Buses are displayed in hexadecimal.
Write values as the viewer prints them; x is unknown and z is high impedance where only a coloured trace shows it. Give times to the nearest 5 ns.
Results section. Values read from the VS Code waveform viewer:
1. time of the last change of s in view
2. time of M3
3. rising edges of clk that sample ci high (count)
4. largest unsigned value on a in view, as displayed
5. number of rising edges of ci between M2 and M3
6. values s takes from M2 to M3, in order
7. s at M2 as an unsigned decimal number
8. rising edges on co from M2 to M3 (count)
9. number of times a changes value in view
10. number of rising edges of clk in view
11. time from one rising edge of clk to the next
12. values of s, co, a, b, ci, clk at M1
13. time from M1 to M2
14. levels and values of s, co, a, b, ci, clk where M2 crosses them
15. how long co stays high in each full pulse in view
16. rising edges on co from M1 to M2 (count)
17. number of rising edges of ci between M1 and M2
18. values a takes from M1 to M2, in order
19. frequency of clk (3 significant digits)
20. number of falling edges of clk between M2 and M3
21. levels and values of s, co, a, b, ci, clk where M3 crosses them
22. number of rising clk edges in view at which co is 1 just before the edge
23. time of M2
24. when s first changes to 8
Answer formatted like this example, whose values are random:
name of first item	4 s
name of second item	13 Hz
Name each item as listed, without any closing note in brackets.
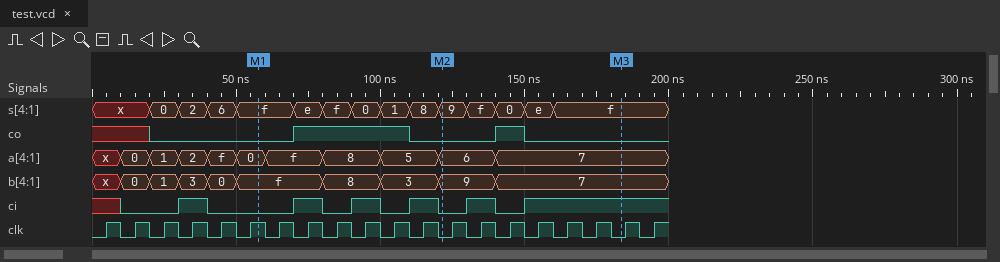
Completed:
time of the last change of s in view	160 ns
time of M3	185 ns
rising edges of clk that sample ci high	10
largest unsigned value on a in view, as displayed	f
number of rising edges of ci between M2 and M3	2
values s takes from M2 to M3, in order	9, f, 0, e, f
s at M2 as an unsigned decimal number	9
rising edges on co from M2 to M3	1
number of times a changes value in view	10
number of rising edges of clk in view	20
time from one rising edge of clk to the next	10 ns
values of s, co, a, b, ci, clk at M1	s=f, co=0, a=0, b=f, ci=0, clk=1
time from M1 to M2	65 ns
levels and values of s, co, a, b, ci, clk where M2 crosses them	s=9, co=0, a=6, b=9, ci=0, clk=0
how long co stays high in each full pulse in view	40 ns, 10 ns
rising edges on co from M1 to M2	1
number of rising edges of ci between M1 and M2	3
values a takes from M1 to M2, in order	0, f, 8, 5, 6
frequency of clk	100 MHz
number of falling edges of clk between M2 and M3	6
levels and values of s, co, a, b, ci, clk where M3 crosses them	s=f, co=0, a=7, b=7, ci=1, clk=0
number of rising clk edges in view at which co is 1 just before the edge	5
time of M2	120 ns
when s first changes to 8	110 ns
